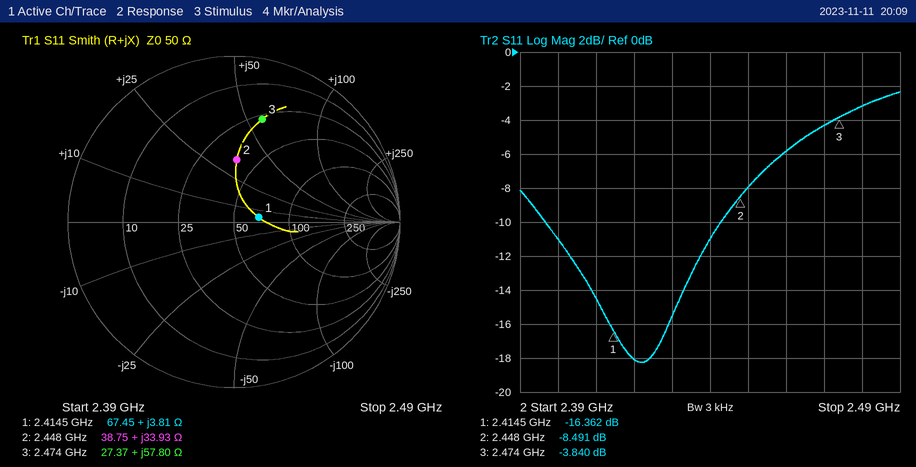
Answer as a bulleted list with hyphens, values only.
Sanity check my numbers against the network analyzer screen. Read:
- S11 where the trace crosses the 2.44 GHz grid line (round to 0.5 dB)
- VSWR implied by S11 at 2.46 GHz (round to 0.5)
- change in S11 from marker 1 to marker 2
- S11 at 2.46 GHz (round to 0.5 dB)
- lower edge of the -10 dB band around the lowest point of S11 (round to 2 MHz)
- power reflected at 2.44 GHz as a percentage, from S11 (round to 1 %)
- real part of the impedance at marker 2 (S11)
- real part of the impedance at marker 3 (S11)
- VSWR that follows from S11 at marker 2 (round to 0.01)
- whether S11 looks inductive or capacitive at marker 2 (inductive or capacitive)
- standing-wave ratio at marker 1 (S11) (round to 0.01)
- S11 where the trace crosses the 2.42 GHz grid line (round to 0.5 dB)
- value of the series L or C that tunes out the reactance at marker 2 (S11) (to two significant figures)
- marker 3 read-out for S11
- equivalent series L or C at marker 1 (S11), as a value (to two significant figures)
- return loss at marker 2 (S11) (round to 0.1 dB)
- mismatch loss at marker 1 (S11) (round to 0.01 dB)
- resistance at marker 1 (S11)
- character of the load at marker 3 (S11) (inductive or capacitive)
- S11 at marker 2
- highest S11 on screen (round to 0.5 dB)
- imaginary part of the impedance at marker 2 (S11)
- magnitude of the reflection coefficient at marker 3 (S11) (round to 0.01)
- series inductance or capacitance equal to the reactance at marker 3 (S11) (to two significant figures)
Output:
- -11.0 dB
- 3.0
- 7.871 dB
- -6.0 dB
- 2.396 GHz
- 8 %
- 38.75 Ω
- 27.37 Ω
- 2.21
- inductive
- 1.36
- -18.0 dB
- 1.9 pF
- -3.840 dB
- 250 pH
- 8.5 dB
- 0.10 dB
- 67.45 Ω
- inductive
- -8.491 dB
- -2.5 dB
- +33.93 Ω
- 0.64
- 3.7 nH
